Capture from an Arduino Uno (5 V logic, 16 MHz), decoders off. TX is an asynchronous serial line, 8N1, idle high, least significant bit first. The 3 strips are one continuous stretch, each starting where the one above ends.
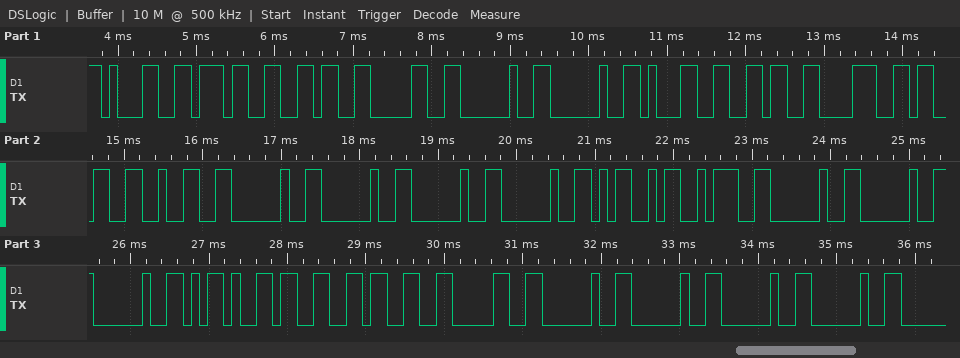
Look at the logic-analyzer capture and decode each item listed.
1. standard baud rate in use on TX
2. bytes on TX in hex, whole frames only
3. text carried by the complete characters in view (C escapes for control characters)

9600 baud
31 37 36 30 20 20 31 36 38 33 32 20 20 20 20 4D 3A 20 20 20 2D 33 33 30 20 20 20 20
"1760  16832    M:   -330    "
